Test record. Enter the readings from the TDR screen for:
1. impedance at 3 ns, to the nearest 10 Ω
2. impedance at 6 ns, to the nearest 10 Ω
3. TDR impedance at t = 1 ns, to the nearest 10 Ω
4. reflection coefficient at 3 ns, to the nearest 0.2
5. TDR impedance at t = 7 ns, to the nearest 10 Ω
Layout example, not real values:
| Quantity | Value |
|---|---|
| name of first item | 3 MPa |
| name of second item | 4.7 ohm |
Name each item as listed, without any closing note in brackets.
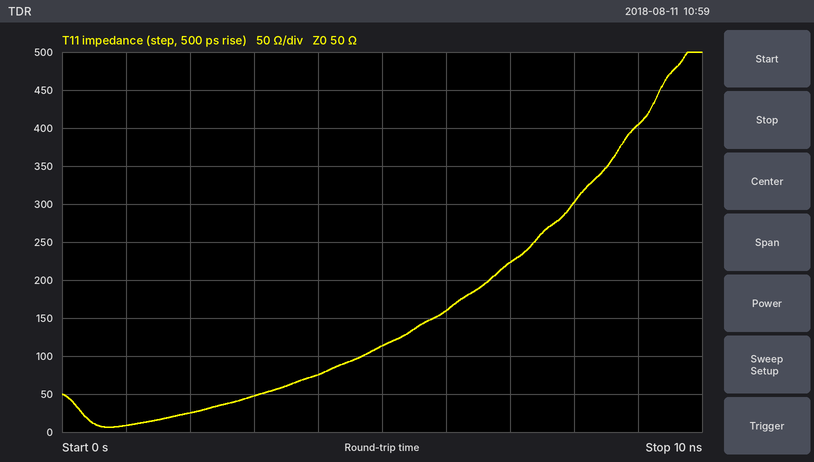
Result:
| Quantity | Value |
|---|---|
| impedance at 3 ns, to the nearest 10 Ω | 50 Ω |
| impedance at 6 ns, to the nearest 10 Ω | 160 Ω |
| TDR impedance at t = 1 ns, to the nearest 10 Ω | 10 Ω |
| reflection coefficient at 3 ns, to the nearest 0.2 | 0.0 |
| TDR impedance at t = 7 ns, to the nearest 10 Ω | 220 Ω |
